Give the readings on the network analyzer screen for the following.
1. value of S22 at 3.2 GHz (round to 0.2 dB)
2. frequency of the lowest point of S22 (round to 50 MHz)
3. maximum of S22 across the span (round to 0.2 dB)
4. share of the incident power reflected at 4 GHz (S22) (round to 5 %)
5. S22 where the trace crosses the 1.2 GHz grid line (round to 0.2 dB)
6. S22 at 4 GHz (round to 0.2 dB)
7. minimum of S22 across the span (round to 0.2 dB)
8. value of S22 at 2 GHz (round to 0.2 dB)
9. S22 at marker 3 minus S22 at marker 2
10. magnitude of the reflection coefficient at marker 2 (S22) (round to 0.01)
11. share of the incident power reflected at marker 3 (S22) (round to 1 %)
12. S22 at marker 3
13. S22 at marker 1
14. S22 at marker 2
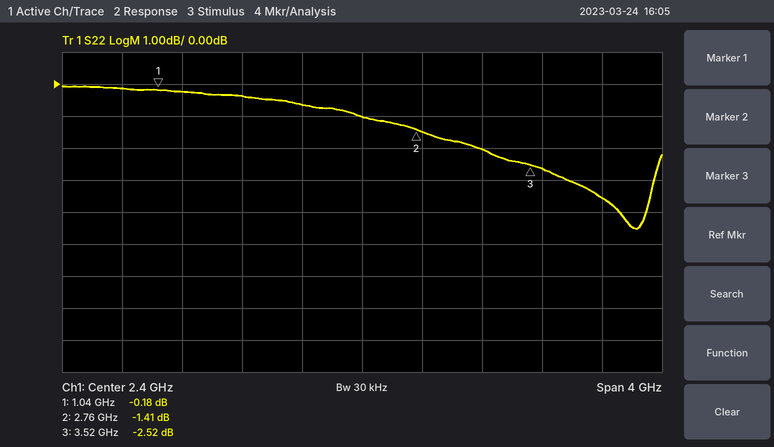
-2.0 dB
4.25 GHz
0.0 dB
45 %
-0.2 dB
-3.6 dB
-4.6 dB
-0.6 dB
-1.11 dB
0.85
56 %
-2.52 dB
-0.18 dB
-1.41 dB
